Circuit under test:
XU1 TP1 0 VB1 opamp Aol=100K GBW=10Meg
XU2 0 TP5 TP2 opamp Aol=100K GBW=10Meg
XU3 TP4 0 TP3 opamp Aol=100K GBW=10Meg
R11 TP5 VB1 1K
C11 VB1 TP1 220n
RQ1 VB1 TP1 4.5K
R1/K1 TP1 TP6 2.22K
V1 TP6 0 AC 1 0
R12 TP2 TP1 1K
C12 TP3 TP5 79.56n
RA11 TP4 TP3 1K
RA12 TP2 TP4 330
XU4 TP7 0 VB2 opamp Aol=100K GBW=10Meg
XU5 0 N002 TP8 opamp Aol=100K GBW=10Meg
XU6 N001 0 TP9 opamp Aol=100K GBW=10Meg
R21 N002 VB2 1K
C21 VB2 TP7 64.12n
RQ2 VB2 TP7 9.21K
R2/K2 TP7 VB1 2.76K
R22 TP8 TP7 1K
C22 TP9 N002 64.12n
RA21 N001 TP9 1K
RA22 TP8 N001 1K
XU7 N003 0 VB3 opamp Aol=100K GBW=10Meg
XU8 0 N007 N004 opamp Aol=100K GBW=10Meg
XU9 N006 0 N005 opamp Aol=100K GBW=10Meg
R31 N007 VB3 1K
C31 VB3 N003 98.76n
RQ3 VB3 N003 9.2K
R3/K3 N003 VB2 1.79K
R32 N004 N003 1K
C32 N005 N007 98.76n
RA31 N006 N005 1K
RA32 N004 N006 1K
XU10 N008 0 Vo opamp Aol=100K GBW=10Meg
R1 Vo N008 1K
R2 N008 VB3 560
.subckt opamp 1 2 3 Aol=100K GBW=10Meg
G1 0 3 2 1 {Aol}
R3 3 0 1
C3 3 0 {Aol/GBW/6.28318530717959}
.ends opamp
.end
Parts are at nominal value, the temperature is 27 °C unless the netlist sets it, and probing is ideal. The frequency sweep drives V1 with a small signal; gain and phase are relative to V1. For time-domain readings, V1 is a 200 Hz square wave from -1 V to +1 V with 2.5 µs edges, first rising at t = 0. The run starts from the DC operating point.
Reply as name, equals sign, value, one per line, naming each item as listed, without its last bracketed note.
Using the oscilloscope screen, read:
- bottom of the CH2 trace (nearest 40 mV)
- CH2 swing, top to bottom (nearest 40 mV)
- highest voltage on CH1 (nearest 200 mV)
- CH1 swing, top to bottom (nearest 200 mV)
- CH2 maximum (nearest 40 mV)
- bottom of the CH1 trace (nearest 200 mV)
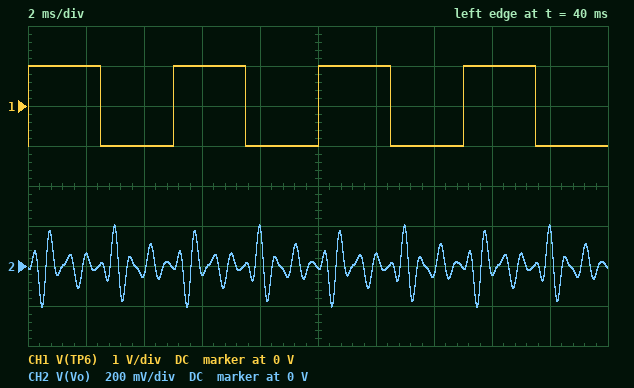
bottom of the CH2 trace = -200 mV
CH2 swing, top to bottom = 400 mV
highest voltage on CH1 = 1.0 V
CH1 swing, top to bottom = 2.0 V
CH2 maximum = 200 mV
bottom of the CH1 trace = -1.0 V
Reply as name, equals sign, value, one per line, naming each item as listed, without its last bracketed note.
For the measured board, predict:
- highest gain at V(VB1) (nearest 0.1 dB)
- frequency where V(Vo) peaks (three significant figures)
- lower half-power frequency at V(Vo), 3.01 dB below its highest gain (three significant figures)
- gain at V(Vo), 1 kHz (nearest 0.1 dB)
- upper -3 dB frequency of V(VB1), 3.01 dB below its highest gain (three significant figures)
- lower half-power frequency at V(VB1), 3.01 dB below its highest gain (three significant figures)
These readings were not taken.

highest gain at V(VB1) = 6.1 dB
frequency where V(Vo) peaks = 1.62 kHz
lower half-power frequency at V(Vo), 3.01 dB below its highest gain = 1.53 kHz
gain at V(Vo), 1 kHz = -19.7 dB
upper -3 dB frequency of V(VB1), 3.01 dB below its highest gain = 776 Hz
lower half-power frequency at V(VB1), 3.01 dB below its highest gain = 615 Hz
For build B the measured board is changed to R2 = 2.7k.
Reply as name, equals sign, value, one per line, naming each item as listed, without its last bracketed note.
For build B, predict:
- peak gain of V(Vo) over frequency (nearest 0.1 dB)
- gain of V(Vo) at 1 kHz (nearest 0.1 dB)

peak gain of V(Vo) over frequency = -14.5 dB
gain of V(Vo) at 1 kHz = -33.3 dB
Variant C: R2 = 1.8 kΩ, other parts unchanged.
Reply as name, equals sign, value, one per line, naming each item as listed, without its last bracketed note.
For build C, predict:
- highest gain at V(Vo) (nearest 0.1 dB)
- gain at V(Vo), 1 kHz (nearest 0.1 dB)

highest gain at V(Vo) = -10.9 dB
gain at V(Vo), 1 kHz = -29.8 dB
